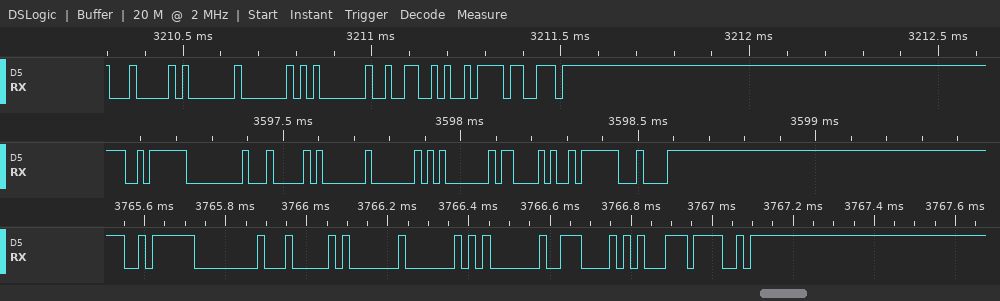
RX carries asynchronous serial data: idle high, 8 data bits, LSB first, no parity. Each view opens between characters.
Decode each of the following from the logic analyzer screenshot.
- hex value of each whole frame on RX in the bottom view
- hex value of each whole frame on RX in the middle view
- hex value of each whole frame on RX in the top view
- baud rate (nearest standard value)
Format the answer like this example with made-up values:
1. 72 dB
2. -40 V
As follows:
1. FA, 00, 04, 01, 40, 01, 0E, C5, 4F
2. FA, 00, 04, 01, 40, 01, 43, FA, 84
3. 04, 01, 40, 01, 32, E9, 73
4. 57600 baud
